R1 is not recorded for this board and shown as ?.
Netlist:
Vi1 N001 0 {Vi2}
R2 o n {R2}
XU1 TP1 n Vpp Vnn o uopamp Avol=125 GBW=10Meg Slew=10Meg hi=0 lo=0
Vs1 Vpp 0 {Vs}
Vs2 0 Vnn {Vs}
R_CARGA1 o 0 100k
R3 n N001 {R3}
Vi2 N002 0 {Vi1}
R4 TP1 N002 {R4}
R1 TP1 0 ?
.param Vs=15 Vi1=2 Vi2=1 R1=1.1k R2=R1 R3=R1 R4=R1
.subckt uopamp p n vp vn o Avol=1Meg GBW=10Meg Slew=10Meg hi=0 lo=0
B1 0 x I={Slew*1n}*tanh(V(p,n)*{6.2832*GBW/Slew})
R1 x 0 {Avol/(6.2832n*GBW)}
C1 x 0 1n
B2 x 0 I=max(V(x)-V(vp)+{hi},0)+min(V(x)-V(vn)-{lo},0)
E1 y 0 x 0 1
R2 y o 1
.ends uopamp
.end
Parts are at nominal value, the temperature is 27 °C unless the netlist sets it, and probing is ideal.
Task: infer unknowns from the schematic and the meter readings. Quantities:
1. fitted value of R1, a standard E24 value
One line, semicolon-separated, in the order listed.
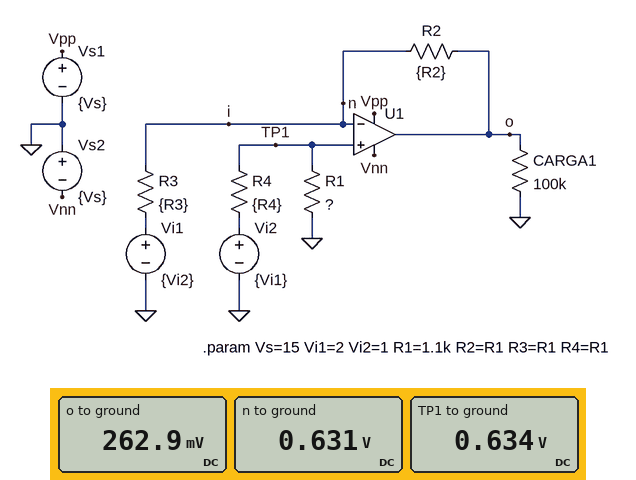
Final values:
510 Ω
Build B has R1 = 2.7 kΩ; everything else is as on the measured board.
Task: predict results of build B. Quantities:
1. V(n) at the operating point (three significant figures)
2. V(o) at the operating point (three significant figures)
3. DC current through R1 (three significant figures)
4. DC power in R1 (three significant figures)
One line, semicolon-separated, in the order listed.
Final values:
1.41 V; 1.81 V; 526 µA; 748 µW
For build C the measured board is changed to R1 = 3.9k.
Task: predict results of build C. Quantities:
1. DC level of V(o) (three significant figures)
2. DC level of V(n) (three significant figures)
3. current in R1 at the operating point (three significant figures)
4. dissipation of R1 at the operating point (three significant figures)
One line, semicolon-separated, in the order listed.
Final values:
2.09 V; 1.54 V; 400 µA; 624 µW
